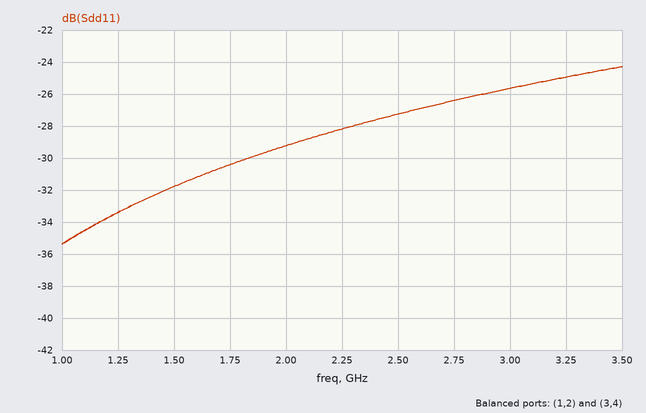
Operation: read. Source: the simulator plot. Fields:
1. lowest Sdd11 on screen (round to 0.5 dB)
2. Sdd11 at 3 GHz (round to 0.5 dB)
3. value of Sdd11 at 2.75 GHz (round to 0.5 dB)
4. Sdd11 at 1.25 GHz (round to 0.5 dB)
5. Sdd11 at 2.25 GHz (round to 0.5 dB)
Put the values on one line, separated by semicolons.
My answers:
-35.5 dB; -25.5 dB; -26.5 dB; -33.5 dB; -28.0 dB
